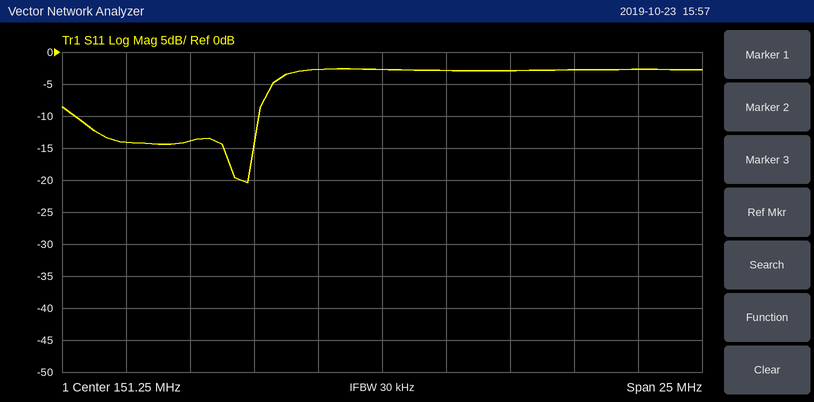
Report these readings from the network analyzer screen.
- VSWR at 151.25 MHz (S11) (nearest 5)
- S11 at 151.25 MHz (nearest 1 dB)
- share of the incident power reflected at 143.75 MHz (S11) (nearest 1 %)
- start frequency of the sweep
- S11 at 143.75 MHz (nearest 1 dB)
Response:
5
-3 dB
4 %
138.75 MHz
-14 dB
